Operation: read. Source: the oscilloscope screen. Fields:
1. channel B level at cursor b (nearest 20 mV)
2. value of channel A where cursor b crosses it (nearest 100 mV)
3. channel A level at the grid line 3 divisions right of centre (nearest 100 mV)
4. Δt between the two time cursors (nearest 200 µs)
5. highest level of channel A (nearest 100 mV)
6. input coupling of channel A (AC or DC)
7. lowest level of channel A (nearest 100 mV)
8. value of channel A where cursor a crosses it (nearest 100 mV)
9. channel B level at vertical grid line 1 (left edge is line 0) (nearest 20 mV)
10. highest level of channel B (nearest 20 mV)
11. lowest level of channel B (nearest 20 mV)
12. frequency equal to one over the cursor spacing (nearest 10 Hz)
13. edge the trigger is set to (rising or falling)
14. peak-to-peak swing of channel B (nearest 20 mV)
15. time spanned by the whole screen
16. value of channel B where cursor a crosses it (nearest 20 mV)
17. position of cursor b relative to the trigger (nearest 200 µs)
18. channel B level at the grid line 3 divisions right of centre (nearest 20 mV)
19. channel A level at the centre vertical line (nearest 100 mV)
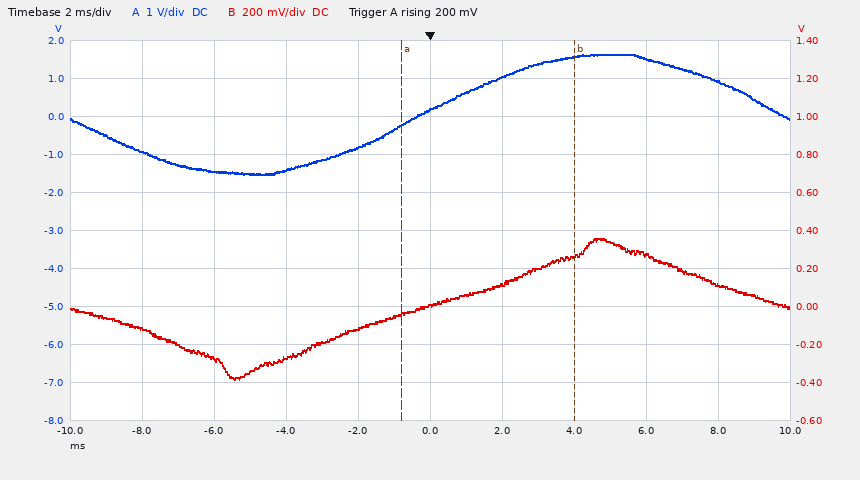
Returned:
260 mV
1.6 V
1.5 V
4.8 ms
1.6 V
DC
-1.5 V
-200 mV
-120 mV
360 mV
-380 mV
210 Hz
rising
740 mV
20 ms
-40 mV
+4.0 ms
280 mV
200 mV
